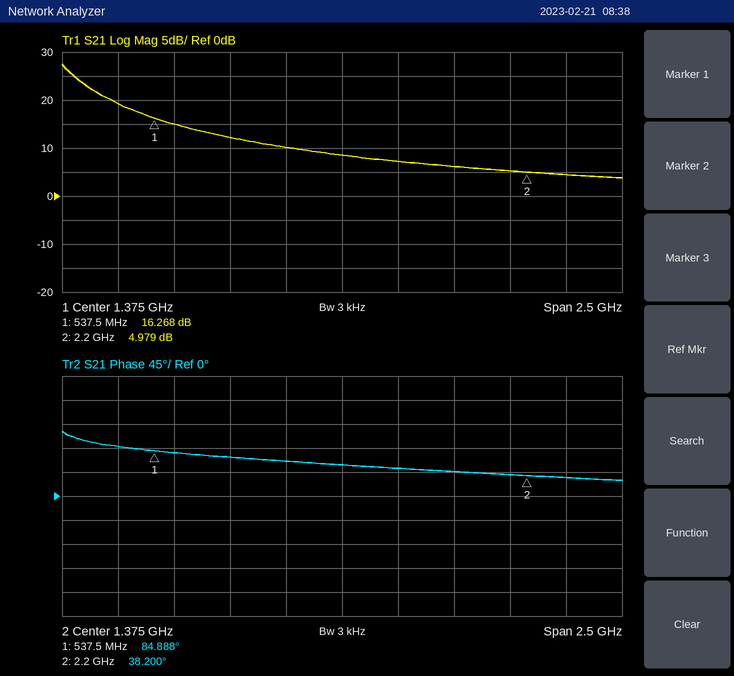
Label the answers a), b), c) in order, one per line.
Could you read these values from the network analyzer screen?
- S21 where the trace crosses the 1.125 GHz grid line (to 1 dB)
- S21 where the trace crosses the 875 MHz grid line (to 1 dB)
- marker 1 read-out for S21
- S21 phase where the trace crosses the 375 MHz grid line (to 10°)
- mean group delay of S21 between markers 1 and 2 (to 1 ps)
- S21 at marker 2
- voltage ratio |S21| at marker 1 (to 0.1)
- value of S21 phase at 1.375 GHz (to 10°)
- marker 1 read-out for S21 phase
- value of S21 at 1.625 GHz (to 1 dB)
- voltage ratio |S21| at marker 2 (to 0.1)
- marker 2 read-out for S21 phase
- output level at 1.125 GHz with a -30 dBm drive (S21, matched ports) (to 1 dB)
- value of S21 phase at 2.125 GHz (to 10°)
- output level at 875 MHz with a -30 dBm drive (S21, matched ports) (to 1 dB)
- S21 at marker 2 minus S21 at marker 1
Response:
a) 10 dB
b) 12 dB
c) 16.268 dB
d) 90°
e) 78 ps
f) 4.979 dB
g) 6.5
h) 60°
i) 84.888°
j) 7 dB
k) 1.8
l) 38.200°
m) -20 dBm
n) 40°
o) -18 dBm
p) -11.289 dB
